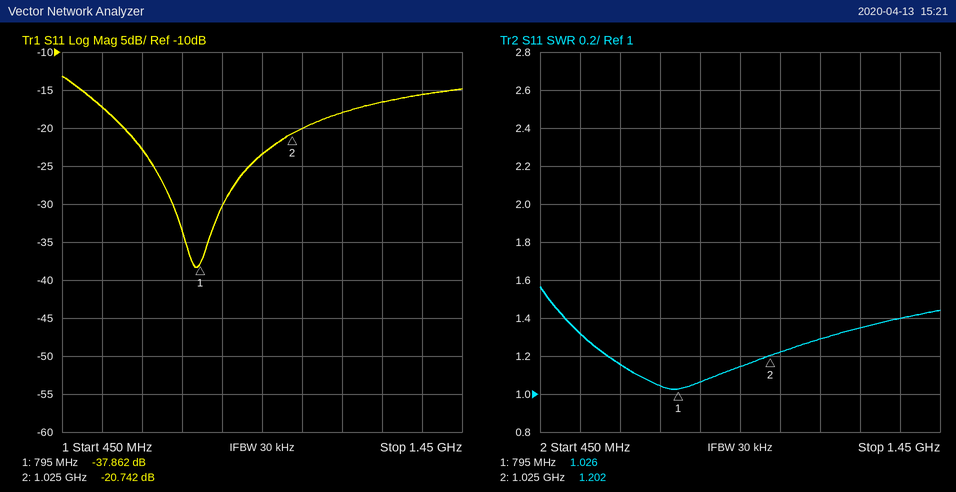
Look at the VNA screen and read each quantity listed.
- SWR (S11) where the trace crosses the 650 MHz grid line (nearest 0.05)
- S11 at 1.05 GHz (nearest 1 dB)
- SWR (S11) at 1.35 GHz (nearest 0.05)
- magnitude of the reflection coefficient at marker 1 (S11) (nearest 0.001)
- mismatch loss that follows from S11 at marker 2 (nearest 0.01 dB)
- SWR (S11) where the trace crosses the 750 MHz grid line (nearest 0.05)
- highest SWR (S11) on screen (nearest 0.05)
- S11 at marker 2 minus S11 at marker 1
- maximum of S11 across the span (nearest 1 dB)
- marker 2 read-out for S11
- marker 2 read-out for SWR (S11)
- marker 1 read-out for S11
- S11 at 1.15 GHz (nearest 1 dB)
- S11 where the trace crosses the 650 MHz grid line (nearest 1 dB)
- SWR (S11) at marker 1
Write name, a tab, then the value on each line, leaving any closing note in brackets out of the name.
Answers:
SWR (S11) where the trace crosses the 650 MHz grid line	1.15
S11 at 1.05 GHz	-20 dB
SWR (S11) at 1.35 GHz	1.40
magnitude of the reflection coefficient at marker 1 (S11)	0.013
mismatch loss that follows from S11 at marker 2	0.04 dB
SWR (S11) where the trace crosses the 750 MHz grid line	1.05
highest SWR (S11) on screen	1.55
S11 at marker 2 minus S11 at marker 1	17.120 dB
maximum of S11 across the span	-13 dB
marker 2 read-out for S11	-20.742 dB
marker 2 read-out for SWR	1.202
marker 1 read-out for S11	-37.862 dB
S11 at 1.15 GHz	-18 dB
S11 where the trace crosses the 650 MHz grid line	-23 dB
SWR (S11) at marker 1	1.026
